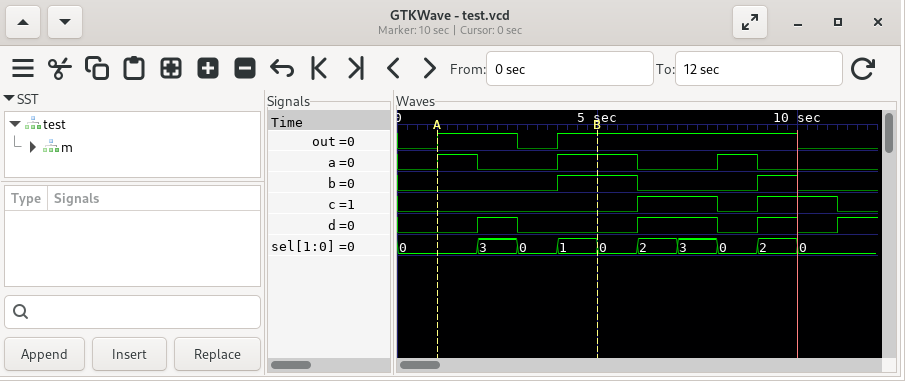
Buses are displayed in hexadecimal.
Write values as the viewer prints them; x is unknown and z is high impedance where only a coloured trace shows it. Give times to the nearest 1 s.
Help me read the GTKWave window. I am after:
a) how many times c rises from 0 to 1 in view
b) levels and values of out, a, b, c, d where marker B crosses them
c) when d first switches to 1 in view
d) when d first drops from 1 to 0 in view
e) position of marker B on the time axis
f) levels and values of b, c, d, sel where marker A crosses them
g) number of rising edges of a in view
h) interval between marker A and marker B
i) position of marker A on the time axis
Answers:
2
out=1, a=1, b=1, c=0, d=0
2 s
3 s
5 s
b=0, c=0, d=0, sel=0
3
4 s
1 s
